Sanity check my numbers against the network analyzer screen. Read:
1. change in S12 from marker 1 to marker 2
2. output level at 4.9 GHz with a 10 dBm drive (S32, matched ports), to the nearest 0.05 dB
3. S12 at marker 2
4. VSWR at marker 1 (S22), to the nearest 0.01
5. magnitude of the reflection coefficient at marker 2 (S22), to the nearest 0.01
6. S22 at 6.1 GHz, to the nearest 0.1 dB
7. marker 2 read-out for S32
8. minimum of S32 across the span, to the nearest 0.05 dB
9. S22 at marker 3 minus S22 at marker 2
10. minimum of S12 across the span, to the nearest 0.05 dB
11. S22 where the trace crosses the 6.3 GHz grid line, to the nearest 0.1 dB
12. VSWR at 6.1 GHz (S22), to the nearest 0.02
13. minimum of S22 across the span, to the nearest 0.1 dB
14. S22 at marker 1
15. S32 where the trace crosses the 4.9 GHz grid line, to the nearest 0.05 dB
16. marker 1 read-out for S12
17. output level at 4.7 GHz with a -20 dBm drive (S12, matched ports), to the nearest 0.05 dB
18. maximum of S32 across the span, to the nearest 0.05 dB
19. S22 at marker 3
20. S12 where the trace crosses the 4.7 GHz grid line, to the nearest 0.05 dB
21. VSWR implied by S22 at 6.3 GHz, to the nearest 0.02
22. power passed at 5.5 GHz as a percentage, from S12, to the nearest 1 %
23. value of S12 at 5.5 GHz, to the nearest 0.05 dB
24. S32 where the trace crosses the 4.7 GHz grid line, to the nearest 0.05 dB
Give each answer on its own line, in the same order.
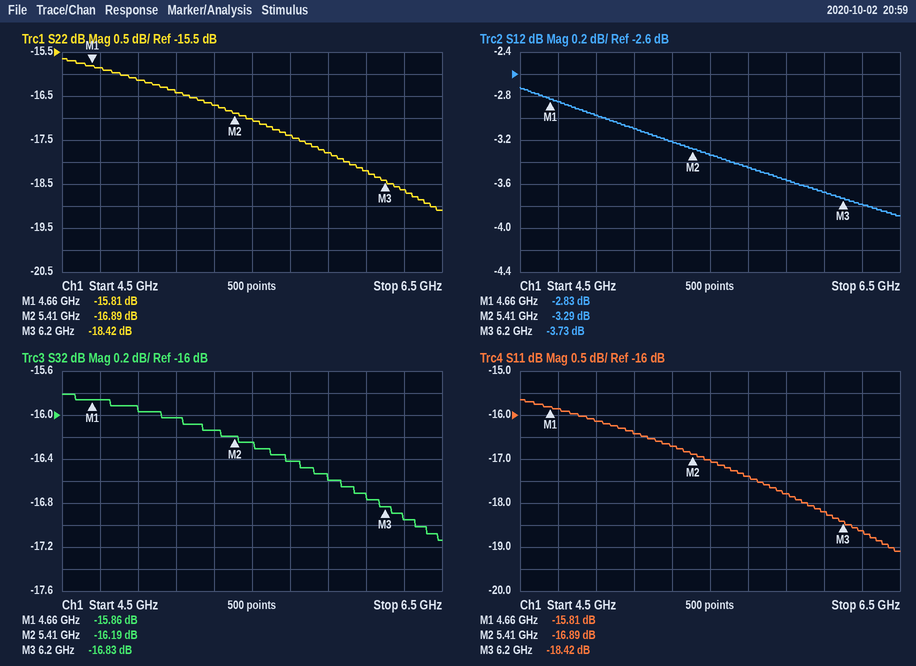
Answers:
-0.46 dB
-5.95 dBm
-3.29 dB
1.39
0.14
-18.2 dB
-16.19 dB
-17.15 dB
-1.53 dB
-3.90 dB
-18.6 dB
1.28
-19.1 dB
-15.81 dB
-15.95 dB
-2.83 dB
-22.85 dBm
-15.80 dB
-18.42 dB
-2.85 dB
1.26
46 %
-3.35 dB
-15.85 dB
